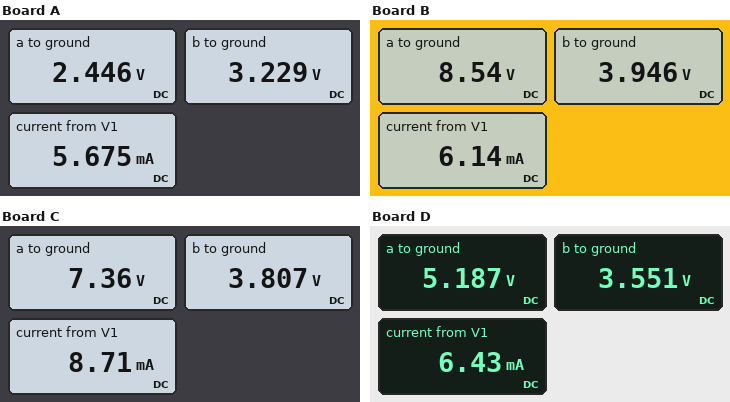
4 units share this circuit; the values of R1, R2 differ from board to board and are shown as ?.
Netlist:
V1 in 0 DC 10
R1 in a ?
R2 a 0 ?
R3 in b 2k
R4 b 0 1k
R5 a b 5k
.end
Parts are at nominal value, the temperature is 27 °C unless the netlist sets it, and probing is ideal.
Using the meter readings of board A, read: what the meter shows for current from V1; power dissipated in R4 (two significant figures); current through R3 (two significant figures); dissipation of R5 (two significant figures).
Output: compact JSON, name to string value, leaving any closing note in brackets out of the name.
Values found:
{"what the meter shows for current from V1": "5.675 mA", "power dissipated in R4": "10 mW", "current through R3": "3.4 mA", "dissipation of R5": "120 µW"}
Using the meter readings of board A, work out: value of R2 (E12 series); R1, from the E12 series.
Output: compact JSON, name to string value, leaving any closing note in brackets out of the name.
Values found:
{"value of R2": "1 kΩ", "R1, from the E12 series": "3.3 kΩ"}
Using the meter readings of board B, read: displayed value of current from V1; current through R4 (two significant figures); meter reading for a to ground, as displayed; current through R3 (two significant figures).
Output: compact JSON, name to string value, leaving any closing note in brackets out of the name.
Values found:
{"displayed value of current from V1": "6.14 mA", "current through R4": "3.9 mA", "meter reading for a to ground, as displayed": "8.54 V", "current through R3": "3.0 mA"}
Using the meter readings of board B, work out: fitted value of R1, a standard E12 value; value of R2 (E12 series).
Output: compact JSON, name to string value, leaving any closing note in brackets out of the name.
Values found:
{"fitted value of R1, a standard E12 value": "470 Ω", "value of R2": "3.9 kΩ"}
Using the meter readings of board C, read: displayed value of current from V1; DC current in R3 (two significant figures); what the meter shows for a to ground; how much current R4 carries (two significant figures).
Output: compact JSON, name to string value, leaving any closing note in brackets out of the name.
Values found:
{"displayed value of current from V1": "8.71 mA", "DC current in R3": "3.1 mA", "what the meter shows for a to ground": "7.36 V", "how much current R4 carries": "3.8 mA"}
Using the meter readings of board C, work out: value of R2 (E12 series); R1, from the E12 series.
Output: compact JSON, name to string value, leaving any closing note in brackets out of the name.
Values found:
{"value of R2": "1.5 kΩ", "R1, from the E12 series": "470 Ω"}
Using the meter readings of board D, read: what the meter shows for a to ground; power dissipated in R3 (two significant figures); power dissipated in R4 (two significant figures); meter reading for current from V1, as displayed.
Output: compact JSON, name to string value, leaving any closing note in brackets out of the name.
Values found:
{"what the meter shows for a to ground": "5.187 V", "power dissipated in R3": "21 mW", "power dissipated in R4": "13 mW", "meter reading for current from V1, as displayed": "6.43 mA"}
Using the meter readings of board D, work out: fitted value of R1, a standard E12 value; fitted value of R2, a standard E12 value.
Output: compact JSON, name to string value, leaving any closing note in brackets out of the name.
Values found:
{"fitted value of R1, a standard E12 value": "1.5 kΩ", "fitted value of R2, a standard E12 value": "1.8 kΩ"}
